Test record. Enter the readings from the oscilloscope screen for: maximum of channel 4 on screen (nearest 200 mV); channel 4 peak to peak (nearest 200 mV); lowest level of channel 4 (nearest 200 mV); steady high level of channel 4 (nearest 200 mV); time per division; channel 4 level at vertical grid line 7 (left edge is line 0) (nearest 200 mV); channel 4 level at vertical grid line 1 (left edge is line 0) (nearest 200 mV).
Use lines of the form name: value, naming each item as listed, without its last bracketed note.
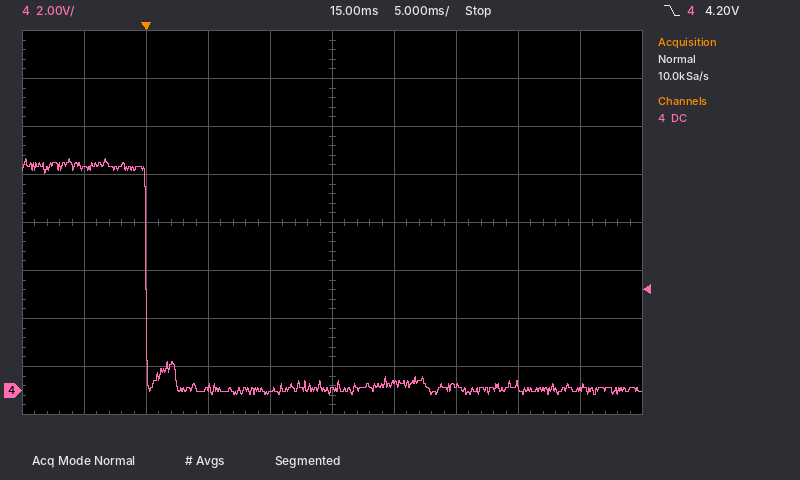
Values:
maximum of channel 4 on screen: 9.6 V
channel 4 peak to peak: 9.8 V
lowest level of channel 4: -200 mV
steady high level of channel 4: 9.4 V
time per division: 5 ms
channel 4 level at vertical grid line 7 (left edge is line 0): 200 mV
channel 4 level at vertical grid line 1 (left edge is line 0): 9.2 V
